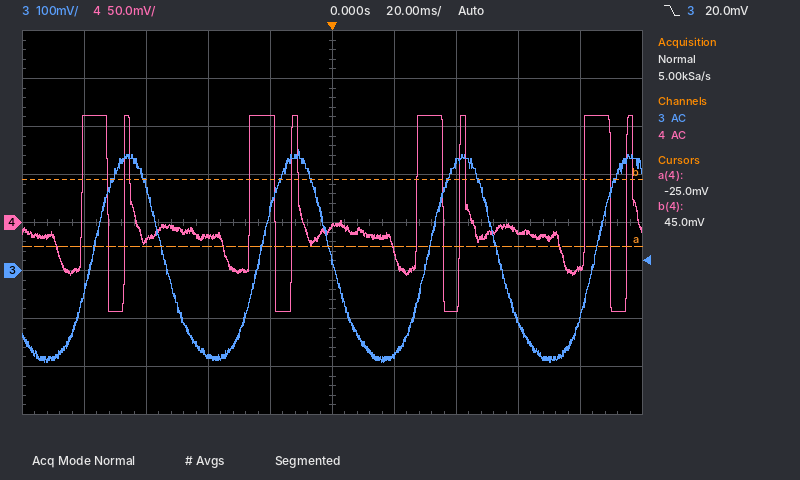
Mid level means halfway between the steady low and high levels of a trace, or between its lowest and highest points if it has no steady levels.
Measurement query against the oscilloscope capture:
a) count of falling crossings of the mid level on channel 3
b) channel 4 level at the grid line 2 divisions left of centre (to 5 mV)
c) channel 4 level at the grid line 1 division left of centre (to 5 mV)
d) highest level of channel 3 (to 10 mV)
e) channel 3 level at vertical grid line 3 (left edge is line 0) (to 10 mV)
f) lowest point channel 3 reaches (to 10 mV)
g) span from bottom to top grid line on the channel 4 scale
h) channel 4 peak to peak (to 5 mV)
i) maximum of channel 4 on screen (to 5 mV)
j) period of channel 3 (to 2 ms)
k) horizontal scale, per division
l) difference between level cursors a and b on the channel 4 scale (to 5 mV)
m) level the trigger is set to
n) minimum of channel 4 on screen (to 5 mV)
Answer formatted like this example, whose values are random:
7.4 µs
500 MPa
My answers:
3
-15 mV
110 mV
250 mV
-180 mV
-190 mV
400 mV
205 mV
110 mV
54 ms
20 ms
70 mV
20.0 mV
-95 mV
